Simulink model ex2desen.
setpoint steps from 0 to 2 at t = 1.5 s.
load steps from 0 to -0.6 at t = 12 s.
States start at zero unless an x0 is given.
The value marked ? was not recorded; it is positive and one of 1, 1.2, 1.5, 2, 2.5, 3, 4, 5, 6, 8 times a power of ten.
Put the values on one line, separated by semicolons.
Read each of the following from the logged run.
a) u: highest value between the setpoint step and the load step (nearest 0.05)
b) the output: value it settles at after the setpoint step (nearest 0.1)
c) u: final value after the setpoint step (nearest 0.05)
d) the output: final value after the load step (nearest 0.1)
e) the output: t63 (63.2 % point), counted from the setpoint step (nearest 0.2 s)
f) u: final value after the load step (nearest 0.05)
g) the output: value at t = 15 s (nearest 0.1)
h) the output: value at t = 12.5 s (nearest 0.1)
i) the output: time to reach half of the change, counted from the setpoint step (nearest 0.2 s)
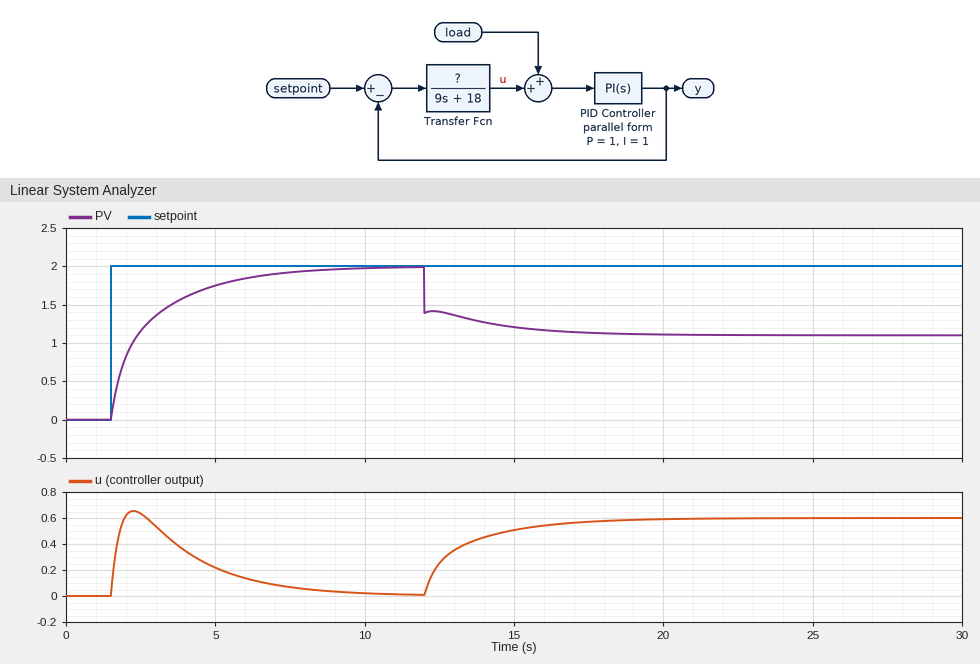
0.65; 2.0; 0.00; 1.1; 1.2 s; 0.60; 1.2; 1.4; 0.8 s
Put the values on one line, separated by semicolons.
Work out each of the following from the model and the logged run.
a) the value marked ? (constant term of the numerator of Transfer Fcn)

12
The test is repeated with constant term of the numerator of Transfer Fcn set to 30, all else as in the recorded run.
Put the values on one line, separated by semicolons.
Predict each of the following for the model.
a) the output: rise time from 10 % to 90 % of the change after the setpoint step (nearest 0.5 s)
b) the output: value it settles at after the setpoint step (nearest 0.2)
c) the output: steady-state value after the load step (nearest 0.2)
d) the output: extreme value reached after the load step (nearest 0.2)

1.5 s; 2.0; 1.6; 1.4
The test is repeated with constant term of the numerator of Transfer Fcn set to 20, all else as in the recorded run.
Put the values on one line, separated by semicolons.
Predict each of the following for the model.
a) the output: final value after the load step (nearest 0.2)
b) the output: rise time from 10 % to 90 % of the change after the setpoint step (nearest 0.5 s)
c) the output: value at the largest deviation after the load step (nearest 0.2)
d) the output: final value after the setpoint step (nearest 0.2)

1.4; 2.5 s; 1.4; 2.0
